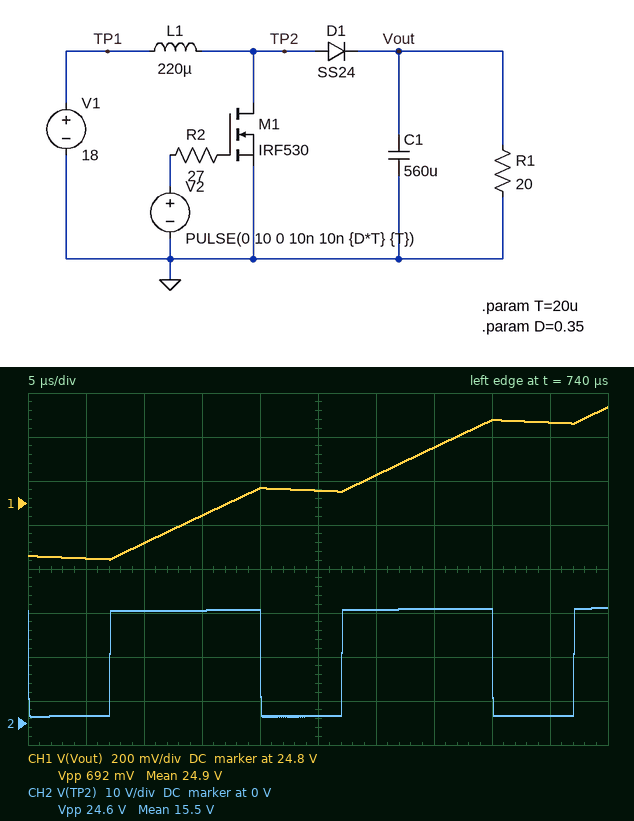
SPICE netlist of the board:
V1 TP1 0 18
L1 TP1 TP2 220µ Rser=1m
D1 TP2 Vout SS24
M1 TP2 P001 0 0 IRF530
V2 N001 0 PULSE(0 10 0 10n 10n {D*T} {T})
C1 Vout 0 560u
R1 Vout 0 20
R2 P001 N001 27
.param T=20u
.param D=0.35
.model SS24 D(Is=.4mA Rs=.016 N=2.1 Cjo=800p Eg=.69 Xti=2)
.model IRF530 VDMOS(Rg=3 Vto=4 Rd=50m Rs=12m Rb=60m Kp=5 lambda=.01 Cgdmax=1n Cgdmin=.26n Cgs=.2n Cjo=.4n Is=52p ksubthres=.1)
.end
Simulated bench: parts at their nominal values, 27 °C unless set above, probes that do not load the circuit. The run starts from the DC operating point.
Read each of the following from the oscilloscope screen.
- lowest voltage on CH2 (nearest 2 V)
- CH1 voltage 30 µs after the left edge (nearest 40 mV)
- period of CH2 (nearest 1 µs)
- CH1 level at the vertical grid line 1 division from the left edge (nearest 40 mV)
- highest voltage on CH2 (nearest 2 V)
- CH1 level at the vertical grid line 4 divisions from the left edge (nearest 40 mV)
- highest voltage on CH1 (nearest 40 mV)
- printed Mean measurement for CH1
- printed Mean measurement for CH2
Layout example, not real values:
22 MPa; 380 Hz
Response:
2 V; 24.92 V; 20 µs; 24.56 V; 26 V; 24.88 V; 25.24 V; 24.9 V; 15.5 V
